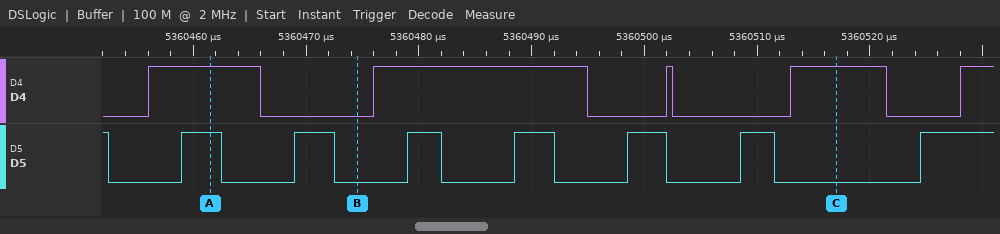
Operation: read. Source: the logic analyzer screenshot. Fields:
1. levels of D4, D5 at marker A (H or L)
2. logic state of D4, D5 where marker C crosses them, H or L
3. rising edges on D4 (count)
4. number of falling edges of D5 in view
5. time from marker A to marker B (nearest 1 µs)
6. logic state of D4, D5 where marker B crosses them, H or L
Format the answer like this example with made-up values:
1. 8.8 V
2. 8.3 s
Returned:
1. D4=H, D5=H
2. D4=H, D5=L
3. 5
4. 7
5. 13 µs
6. D4=L, D5=L
